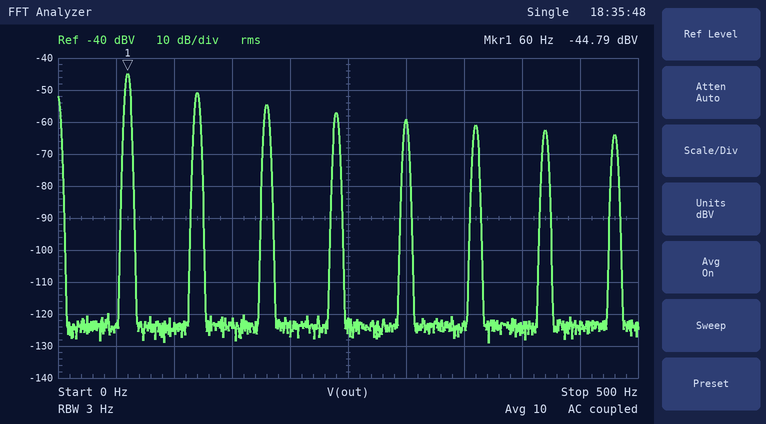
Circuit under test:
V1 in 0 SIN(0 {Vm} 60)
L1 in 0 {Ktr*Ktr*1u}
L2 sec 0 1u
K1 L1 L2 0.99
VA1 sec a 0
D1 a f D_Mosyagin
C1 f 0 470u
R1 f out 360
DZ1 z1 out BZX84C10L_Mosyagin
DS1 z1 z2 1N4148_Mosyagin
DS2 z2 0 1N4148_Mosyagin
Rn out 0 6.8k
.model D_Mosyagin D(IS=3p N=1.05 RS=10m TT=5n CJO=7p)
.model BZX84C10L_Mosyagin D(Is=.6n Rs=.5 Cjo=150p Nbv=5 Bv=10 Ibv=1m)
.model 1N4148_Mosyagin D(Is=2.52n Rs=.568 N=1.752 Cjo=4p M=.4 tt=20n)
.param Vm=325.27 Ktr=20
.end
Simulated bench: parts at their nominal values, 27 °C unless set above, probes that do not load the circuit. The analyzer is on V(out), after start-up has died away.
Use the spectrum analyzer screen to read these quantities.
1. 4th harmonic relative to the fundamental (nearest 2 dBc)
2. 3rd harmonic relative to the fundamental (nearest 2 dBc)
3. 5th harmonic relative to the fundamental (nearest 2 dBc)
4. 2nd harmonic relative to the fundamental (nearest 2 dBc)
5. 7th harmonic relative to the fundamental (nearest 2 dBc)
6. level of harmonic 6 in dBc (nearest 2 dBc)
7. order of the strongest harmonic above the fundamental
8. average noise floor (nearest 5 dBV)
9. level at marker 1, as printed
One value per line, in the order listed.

-12 dBc
-10 dBc
-14 dBc
-6 dBc
-18 dBc
-16 dBc
2
-125 dBV
-44.79 dBV
